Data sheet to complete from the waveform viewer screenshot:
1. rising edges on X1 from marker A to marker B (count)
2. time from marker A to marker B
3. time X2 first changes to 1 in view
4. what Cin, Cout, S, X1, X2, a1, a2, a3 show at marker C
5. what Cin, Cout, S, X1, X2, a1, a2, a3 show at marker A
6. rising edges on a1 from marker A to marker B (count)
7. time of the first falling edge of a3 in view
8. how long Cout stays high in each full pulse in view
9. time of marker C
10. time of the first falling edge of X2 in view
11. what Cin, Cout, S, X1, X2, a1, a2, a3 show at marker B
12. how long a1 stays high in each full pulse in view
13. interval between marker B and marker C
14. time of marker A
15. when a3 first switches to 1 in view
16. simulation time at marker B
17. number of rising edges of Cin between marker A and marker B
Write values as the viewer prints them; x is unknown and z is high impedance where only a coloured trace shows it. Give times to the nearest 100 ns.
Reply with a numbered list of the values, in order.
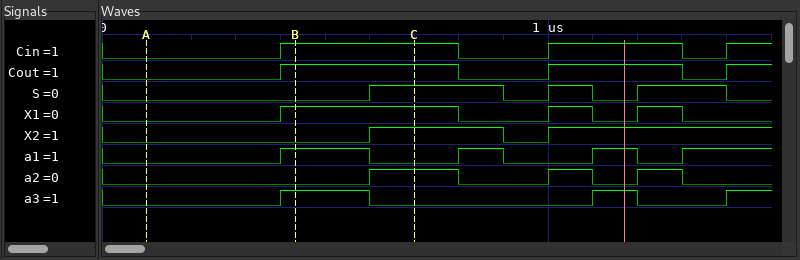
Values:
1. 1
2. 300 ns
3. 600 ns
4. Cin=1, Cout=1, S=1, X1=1, X2=1, a1=0, a2=1, a3=0
5. Cin=0, Cout=0, S=0, X1=0, X2=0, a1=0, a2=0, a3=0
6. 1
7. 600 ns
8. 400 ns, 300 ns
9. 700 ns
10. 900 ns
11. Cin=1, Cout=1, S=0, X1=1, X2=0, a1=1, a2=0, a3=1
12. 200 ns, 100 ns, 100 ns
13. 300 ns
14. 100 ns
15. 400 ns
16. 400 ns
17. 1
